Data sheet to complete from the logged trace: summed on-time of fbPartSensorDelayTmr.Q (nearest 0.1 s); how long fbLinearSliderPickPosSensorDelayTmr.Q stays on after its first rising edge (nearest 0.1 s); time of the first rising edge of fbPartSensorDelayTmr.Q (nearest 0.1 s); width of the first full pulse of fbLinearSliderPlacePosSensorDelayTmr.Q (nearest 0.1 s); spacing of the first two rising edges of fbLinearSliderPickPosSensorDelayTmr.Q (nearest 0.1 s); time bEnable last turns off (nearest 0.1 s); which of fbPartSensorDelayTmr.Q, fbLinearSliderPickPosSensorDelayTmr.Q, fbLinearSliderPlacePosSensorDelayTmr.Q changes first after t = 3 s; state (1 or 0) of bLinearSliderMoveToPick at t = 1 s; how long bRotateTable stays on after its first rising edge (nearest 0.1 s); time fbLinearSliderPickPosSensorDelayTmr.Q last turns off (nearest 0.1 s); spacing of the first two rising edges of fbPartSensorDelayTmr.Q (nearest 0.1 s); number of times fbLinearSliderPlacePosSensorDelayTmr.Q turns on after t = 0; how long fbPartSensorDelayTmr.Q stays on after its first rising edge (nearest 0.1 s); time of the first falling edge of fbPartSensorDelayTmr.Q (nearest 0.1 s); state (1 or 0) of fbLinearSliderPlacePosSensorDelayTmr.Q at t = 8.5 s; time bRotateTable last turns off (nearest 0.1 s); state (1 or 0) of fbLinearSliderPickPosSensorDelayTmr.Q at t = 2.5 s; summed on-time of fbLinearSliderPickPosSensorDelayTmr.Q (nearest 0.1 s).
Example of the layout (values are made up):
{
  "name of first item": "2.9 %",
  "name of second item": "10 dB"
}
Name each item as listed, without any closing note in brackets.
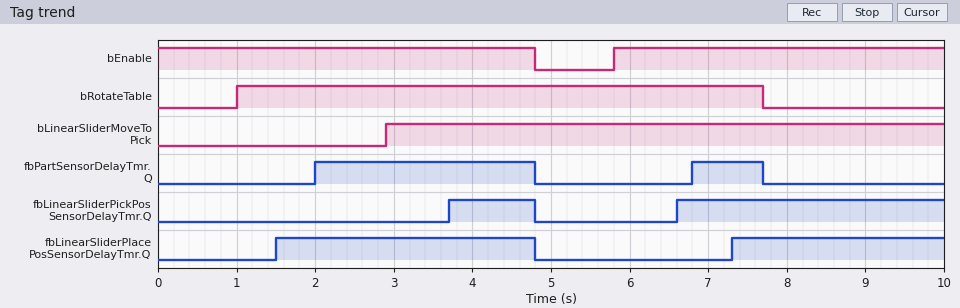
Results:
{
  "summed on-time of fbPartSensorDelayTmr.Q": "3.7 s",
  "how long fbLinearSliderPickPosSensorDelayTmr.Q stays on after its first rising edge": "1.1 s",
  "time of the first rising edge of fbPartSensorDelayTmr.Q": "2.0 s",
  "width of the first full pulse of fbLinearSliderPlacePosSensorDelayTmr.Q": "3.3 s",
  "spacing of the first two rising edges of fbLinearSliderPickPosSensorDelayTmr.Q": "2.9 s",
  "time bEnable last turns off": "4.8 s",
  "which of fbPartSensorDelayTmr.Q, fbLinearSliderPickPosSensorDelayTmr.Q, fbLinearSliderPlacePosSensorDelayTmr.Q changes first after t = 3 s": "fbLinearSliderPickPosSensorDelayTmr.Q",
  "state (1 or 0) of bLinearSliderMoveToPick at t = 1 s": "0",
  "how long bRotateTable stays on after its first rising edge": "6.7 s",
  "time fbLinearSliderPickPosSensorDelayTmr.Q last turns off": "4.8 s",
  "spacing of the first two rising edges of fbPartSensorDelayTmr.Q": "4.8 s",
  "number of times fbLinearSliderPlacePosSensorDelayTmr.Q turns on after t = 0": "2",
  "how long fbPartSensorDelayTmr.Q stays on after its first rising edge": "2.8 s",
  "time of the first falling edge of fbPartSensorDelayTmr.Q": "4.8 s",
  "state (1 or 0) of fbLinearSliderPlacePosSensorDelayTmr.Q at t = 8.5 s": "1",
  "time bRotateTable last turns off": "7.7 s",
  "state (1 or 0) of fbLinearSliderPickPosSensorDelayTmr.Q at t = 2.5 s": "0",
  "summed on-time of fbLinearSliderPickPosSensorDelayTmr.Q": "4.5 s"
}
